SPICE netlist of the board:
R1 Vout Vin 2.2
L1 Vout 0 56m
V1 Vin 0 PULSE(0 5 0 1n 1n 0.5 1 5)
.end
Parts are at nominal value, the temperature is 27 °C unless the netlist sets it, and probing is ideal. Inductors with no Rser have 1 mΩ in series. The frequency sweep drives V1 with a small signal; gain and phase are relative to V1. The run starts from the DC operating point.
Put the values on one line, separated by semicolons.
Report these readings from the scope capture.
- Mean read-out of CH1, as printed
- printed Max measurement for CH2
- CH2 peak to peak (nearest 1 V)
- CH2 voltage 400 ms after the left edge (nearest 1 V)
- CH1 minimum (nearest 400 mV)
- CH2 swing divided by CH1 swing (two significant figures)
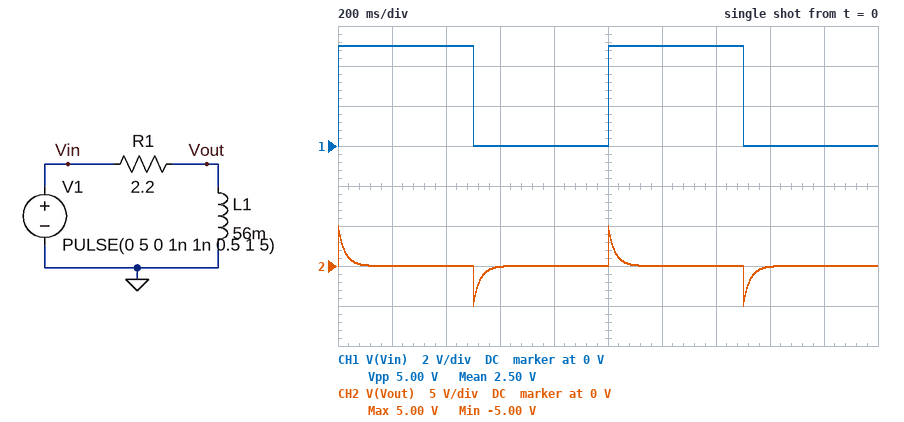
2.50 V; 5.00 V; 10 V; 0 V; 0 V; 2.0
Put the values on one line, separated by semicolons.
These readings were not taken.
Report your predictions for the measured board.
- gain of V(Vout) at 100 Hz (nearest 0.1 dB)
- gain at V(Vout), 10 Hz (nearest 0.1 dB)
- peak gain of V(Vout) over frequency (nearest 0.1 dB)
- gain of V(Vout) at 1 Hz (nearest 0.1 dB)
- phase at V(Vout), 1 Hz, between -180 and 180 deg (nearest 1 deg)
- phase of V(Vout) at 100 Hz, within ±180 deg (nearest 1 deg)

0 dB; -1.4 dB; 0 dB; -16.0 dB; 81 deg; 4 deg
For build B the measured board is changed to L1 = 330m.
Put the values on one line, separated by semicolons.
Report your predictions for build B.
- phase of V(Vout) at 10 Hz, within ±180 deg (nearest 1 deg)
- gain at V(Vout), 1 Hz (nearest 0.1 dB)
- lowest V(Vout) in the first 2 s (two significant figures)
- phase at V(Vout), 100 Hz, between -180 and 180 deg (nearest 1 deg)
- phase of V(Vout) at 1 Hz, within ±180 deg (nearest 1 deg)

6 deg; -3.3 dB; -4.8 V; 1 deg; 47 deg
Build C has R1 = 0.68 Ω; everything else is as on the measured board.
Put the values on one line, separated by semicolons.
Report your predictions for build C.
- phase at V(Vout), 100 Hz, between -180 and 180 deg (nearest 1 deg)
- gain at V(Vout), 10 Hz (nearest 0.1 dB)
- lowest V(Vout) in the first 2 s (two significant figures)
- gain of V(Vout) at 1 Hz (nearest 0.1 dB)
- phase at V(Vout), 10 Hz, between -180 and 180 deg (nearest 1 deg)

1 deg; -0.2 dB; -5.0 V; -6.8 dB; 11 deg
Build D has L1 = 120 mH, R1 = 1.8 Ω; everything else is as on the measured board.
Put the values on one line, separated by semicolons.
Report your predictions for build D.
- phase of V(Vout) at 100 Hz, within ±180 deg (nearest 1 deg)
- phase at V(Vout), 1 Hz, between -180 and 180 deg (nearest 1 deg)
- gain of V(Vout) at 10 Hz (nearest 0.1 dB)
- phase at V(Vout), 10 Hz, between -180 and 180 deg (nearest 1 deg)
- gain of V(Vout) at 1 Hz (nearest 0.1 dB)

1 deg; 67 deg; -0.2 dB; 13 deg; -8.3 dB
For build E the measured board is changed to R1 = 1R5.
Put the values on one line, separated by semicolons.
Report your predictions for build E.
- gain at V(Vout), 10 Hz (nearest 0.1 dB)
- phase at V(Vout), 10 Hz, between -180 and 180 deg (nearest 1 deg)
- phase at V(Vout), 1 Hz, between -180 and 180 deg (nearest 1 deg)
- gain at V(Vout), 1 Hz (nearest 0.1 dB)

-0.7 dB; 23 deg; 77 deg; -12.8 dB
